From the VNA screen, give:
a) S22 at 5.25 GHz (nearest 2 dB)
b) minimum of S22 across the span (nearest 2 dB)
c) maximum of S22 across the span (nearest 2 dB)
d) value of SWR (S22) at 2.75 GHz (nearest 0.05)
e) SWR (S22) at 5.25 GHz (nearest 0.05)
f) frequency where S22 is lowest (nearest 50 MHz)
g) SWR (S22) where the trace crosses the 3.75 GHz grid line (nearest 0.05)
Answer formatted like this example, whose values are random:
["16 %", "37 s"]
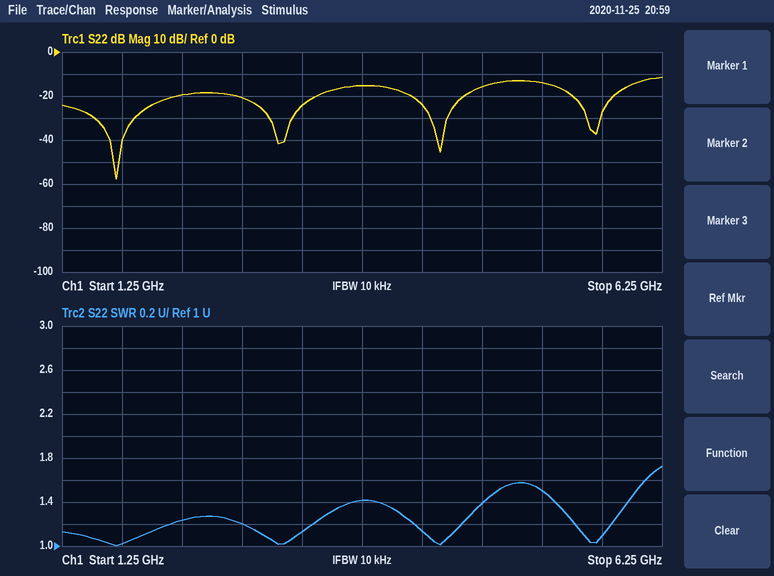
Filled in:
["-14 dB", "-58 dB", "-12 dB", "1.20", "1.50", "1.70 GHz", "1.40"]
